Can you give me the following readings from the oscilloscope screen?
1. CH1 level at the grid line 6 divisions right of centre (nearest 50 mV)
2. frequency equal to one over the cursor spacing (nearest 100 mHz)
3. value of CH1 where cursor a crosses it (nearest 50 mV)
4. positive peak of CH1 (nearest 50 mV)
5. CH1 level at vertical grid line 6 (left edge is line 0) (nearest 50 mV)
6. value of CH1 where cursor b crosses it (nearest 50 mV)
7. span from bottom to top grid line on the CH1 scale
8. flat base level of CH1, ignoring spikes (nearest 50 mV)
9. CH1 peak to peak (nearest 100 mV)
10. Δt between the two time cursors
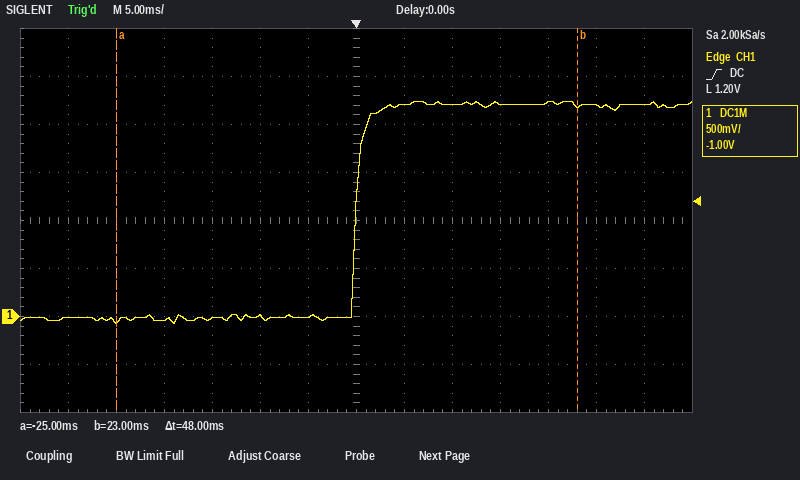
2.20 V
20.8 Hz
-50 mV
2.25 V
0 mV
2.20 V
4 V
0 mV
2.30 V
48 ms
